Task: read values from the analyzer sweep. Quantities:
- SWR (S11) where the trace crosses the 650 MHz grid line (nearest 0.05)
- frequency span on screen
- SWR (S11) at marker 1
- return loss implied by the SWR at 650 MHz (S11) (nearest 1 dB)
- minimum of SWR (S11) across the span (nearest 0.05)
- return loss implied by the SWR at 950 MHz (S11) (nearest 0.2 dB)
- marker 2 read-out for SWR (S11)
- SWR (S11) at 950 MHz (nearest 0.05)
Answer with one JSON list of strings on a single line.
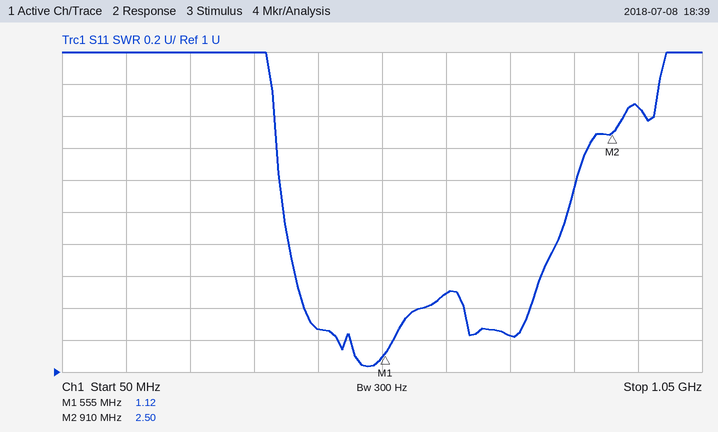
["1.50", "1 GHz", "1.12", "14 dB", "1.05", "6.8 dB", "2.50", "2.65"]
